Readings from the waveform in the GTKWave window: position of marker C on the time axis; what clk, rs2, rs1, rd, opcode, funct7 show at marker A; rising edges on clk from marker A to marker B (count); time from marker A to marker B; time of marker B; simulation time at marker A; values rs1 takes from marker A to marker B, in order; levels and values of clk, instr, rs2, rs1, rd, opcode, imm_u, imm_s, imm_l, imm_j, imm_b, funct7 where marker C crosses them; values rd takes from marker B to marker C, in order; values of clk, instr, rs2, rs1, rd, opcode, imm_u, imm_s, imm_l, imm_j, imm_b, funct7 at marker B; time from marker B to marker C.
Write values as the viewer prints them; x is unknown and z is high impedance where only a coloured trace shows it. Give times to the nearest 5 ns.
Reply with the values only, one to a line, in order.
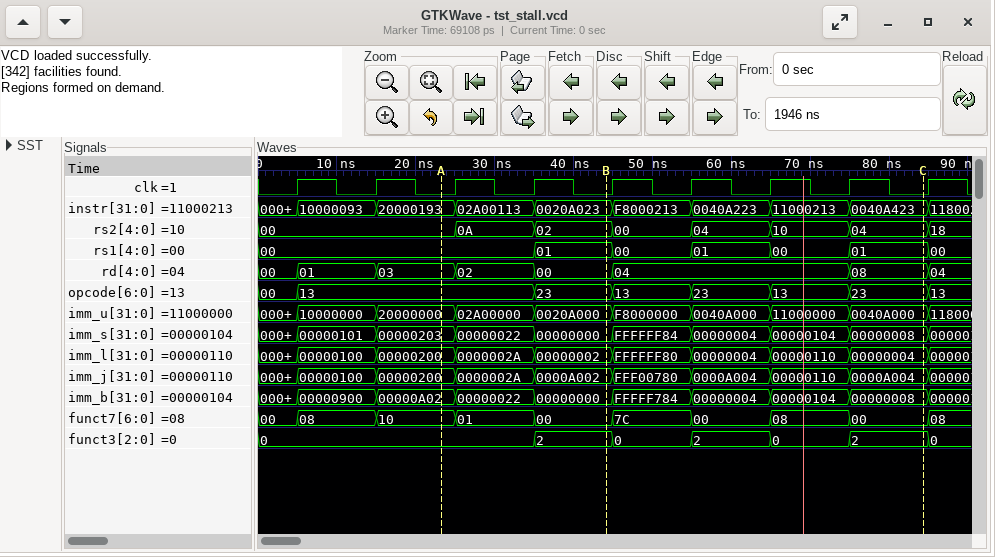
85 ns
clk=0, rs2=00, rs1=00, rd=03, opcode=13, funct7=10
2
20 ns
45 ns
25 ns
00, 01
clk=0, instr=0040A423, rs2=04, rs1=01, rd=08, opcode=23, imm_u=0040A000, imm_s=00000008, imm_l=00000004, imm_j=0000A004, imm_b=00000008, funct7=00
00, 04, 08
clk=0, instr=0020A023, rs2=02, rs1=01, rd=00, opcode=23, imm_u=0020A000, imm_s=00000000, imm_l=00000002, imm_j=0000A002, imm_b=00000000, funct7=00
40 ns
